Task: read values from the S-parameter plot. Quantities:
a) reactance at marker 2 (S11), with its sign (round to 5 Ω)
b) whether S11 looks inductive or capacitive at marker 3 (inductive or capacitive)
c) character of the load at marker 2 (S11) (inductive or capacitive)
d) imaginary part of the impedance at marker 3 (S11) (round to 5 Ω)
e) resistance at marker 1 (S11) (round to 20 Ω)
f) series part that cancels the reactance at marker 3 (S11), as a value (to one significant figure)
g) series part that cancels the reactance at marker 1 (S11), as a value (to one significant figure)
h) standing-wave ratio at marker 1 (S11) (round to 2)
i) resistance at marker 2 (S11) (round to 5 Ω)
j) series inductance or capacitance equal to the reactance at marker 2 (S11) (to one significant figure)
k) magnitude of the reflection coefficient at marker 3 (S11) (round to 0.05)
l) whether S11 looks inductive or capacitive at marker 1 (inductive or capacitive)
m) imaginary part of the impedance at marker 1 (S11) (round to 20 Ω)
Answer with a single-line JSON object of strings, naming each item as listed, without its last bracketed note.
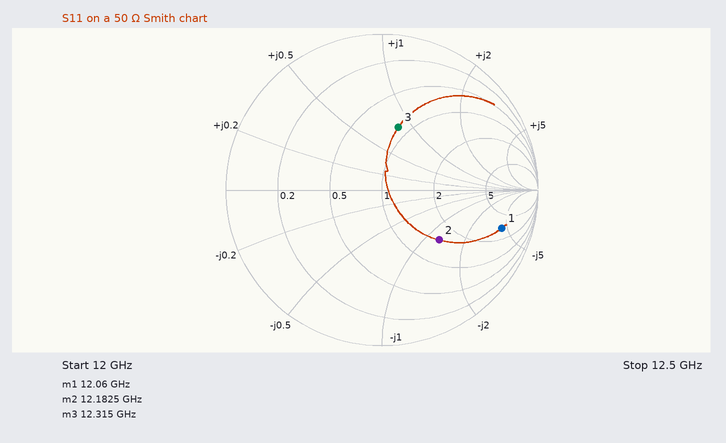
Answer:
{"reactance at marker 2 (S11), with its sign": "-65 Ω", "whether S11 looks inductive or capacitive at marker 3": "inductive", "character of the load at marker 2 (S11)": "capacitive", "imaginary part of the impedance at marker 3 (S11)": "+40 Ω", "resistance at marker 1 (S11)": "160 Ω", "series part that cancels the reactance at marker 3 (S11), as a value": "300 fF", "series part that cancels the reactance at marker 1 (S11), as a value": "3 nH", "standing-wave ratio at marker 1 (S11)": "10", "resistance at marker 2 (S11)": "75 Ω", "series inductance or capacitance equal to the reactance at marker 2 (S11)": "200 fF", "magnitude of the reflection coefficient at marker 3 (S11)": "0.40", "whether S11 looks inductive or capacitive at marker 1": "capacitive", "imaginary part of the impedance at marker 1 (S11)": "-220 Ω"}
